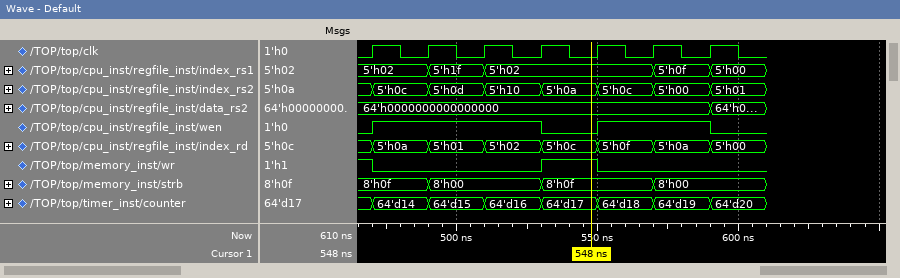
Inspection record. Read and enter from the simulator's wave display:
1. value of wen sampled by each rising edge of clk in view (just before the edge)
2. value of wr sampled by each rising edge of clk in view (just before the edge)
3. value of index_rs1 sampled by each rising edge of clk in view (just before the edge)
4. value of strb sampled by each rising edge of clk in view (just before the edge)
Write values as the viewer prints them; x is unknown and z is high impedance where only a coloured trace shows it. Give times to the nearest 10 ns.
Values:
0 1 1 1 0 1 1
1 0 0 0 1 0 0
5'h02, 5'h02, 5'h1f, 5'h02, 5'h02, 5'h02, 5'h0f
8'h0f, 8'h0f, 8'h00, 8'h00, 8'h0f, 8'h0f, 8'h00
